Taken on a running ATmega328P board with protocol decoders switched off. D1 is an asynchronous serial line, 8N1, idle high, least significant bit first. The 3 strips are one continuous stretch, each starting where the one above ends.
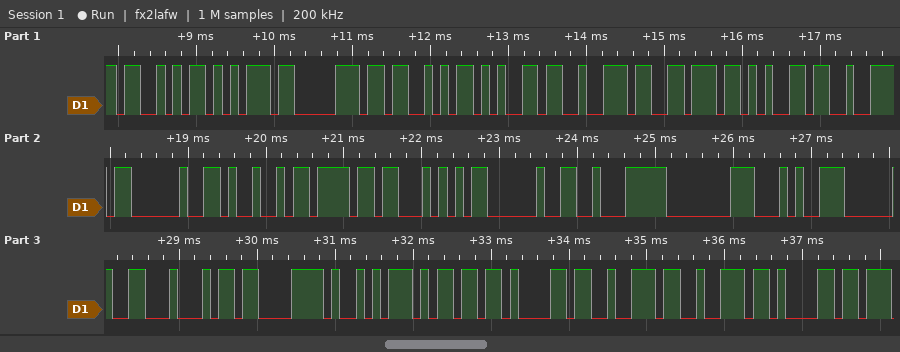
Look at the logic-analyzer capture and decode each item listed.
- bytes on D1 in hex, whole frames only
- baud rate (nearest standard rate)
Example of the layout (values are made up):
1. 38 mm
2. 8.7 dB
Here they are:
1. 53 75 70 53 65 72 76 65 72 20 49 6F 54 20 E2 80 94 20 44 C3 A9 6D 61 72 72 61
2. 9600 baud
